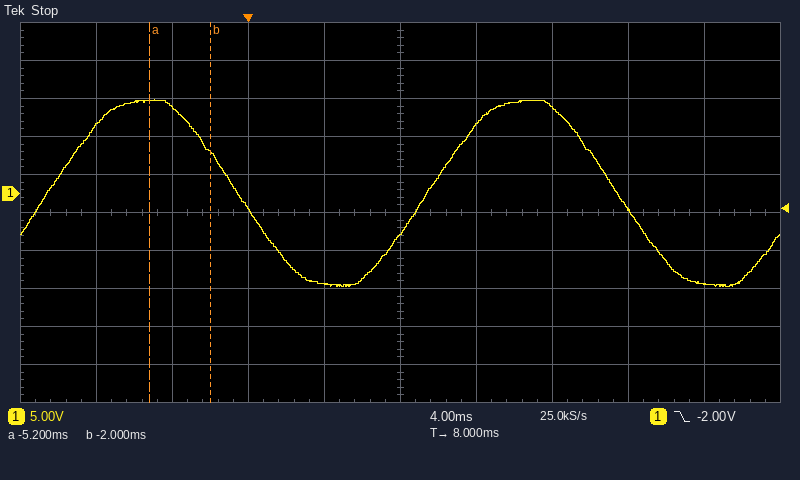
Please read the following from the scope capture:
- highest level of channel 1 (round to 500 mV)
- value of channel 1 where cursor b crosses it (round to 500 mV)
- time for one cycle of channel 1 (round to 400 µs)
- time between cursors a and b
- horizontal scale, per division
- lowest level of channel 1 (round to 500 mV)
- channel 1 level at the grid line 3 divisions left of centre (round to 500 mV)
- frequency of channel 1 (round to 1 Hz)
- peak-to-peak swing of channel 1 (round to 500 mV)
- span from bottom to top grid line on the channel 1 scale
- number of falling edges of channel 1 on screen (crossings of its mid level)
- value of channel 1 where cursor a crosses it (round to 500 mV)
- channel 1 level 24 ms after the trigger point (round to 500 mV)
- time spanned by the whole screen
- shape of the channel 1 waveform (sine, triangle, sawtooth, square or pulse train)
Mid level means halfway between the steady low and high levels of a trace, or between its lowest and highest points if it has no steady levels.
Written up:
12.5 V
5.5 V
20.0 ms
3.2 ms
4 ms
-12.0 V
11.5 V
50 Hz
24.5 V
50 V
2
12.0 V
-12.0 V
40 ms
sine
